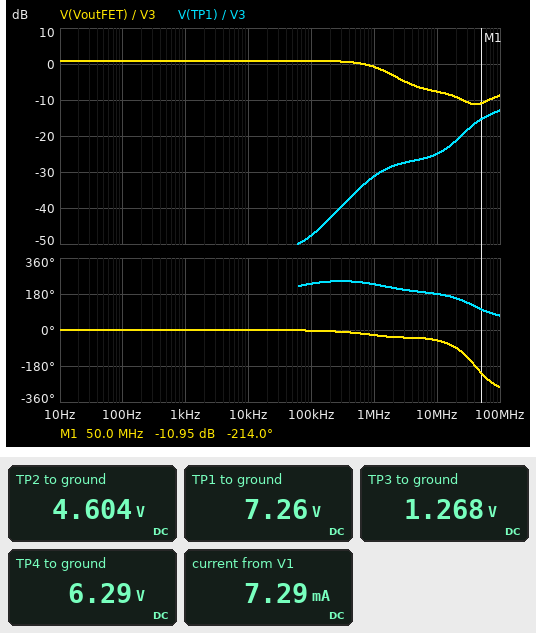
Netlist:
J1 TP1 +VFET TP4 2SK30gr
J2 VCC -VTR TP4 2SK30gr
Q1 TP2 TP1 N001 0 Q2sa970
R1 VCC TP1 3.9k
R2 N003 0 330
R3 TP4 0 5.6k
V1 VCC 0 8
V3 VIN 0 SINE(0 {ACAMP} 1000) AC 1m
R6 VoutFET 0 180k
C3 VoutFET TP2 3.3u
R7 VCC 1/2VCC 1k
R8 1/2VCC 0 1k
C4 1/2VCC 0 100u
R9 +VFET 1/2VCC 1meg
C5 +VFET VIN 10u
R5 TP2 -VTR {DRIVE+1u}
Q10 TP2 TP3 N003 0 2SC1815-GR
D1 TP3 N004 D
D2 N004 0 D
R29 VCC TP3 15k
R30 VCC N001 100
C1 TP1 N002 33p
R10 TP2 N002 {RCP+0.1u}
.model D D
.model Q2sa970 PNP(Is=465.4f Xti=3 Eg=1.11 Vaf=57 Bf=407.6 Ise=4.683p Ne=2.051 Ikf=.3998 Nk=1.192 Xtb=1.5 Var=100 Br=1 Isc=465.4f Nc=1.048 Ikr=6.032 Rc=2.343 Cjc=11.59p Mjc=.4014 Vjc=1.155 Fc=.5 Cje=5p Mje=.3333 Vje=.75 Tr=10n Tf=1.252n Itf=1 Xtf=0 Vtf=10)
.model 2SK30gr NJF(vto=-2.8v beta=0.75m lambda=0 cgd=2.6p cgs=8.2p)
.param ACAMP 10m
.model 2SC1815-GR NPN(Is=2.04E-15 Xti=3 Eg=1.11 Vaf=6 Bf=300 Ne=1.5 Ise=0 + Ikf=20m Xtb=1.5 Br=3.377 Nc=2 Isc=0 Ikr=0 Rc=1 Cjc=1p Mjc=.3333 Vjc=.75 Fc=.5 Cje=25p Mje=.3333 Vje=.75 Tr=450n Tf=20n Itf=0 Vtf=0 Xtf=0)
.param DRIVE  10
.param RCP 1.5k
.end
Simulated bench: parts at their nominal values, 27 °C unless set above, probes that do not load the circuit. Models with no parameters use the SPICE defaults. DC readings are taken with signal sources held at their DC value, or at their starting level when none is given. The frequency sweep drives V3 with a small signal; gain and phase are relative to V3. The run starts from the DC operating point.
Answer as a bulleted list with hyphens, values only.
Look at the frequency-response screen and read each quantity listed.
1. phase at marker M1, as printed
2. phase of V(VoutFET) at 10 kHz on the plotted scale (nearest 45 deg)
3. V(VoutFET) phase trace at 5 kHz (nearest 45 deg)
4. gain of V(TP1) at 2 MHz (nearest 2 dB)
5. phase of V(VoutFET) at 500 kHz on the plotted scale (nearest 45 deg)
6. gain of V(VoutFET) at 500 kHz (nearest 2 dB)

- -214.0 deg
- 0 deg
- 0 deg
- -28 dB
- 0 deg
- 0 dB
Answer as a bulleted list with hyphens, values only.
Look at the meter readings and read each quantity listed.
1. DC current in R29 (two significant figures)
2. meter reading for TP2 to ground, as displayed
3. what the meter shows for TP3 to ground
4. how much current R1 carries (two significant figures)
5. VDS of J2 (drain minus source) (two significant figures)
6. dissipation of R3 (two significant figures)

- 450 µA
- 4.604 V
- 1.268 V
- 190 µA
- 1.7 V
- 7.1 mW
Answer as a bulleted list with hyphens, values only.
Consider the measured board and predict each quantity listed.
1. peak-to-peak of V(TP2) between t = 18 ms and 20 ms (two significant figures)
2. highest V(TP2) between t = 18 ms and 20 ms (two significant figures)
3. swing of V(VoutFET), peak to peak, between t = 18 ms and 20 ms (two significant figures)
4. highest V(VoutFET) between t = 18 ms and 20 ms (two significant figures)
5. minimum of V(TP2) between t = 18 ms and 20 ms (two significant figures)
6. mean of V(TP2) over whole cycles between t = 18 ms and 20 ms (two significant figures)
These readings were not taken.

- 22 mV
- 4.6 V
- 22 mV
- 11 mV
- 4.6 V
- 4.6 V
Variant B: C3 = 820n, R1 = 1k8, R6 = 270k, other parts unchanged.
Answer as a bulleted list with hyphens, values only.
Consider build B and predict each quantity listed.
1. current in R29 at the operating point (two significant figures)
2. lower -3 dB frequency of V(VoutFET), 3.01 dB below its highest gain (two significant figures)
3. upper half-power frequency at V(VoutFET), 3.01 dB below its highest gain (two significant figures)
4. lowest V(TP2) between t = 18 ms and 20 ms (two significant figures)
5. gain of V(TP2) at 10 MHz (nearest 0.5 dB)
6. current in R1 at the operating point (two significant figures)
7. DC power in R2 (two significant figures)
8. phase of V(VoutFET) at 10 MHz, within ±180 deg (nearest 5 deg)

- 450 µA
- 720 mHz
- 1.7 MHz
- 4.2 V
- -7.0 dB
- 410 µA
- 970 µW
- -45 deg
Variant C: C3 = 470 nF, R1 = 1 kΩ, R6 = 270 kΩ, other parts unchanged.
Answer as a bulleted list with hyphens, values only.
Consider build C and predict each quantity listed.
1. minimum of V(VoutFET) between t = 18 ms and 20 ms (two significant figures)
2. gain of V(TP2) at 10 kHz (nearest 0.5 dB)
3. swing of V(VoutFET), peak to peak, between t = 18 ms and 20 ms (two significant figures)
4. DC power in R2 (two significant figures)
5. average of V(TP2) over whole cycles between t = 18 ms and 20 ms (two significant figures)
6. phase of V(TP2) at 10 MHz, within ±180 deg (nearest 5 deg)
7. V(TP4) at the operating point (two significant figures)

- -12 mV
- 1.5 dB
- 24 mV
- 970 µW
- 3.6 V
- -45 deg
- 5.8 V
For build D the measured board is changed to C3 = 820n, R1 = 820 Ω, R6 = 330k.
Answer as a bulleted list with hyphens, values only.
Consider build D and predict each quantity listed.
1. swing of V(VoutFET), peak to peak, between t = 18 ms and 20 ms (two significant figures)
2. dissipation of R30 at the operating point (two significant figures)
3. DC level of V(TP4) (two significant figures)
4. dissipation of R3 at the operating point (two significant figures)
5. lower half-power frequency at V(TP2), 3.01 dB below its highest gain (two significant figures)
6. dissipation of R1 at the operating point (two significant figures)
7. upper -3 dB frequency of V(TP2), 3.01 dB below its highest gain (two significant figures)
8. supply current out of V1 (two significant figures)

- 26 mV
- 290 µW
- 5.7 V
- 5.8 mW
- 16 mHz
- 670 µW
- 1.1 MHz
- 7.2 mA
